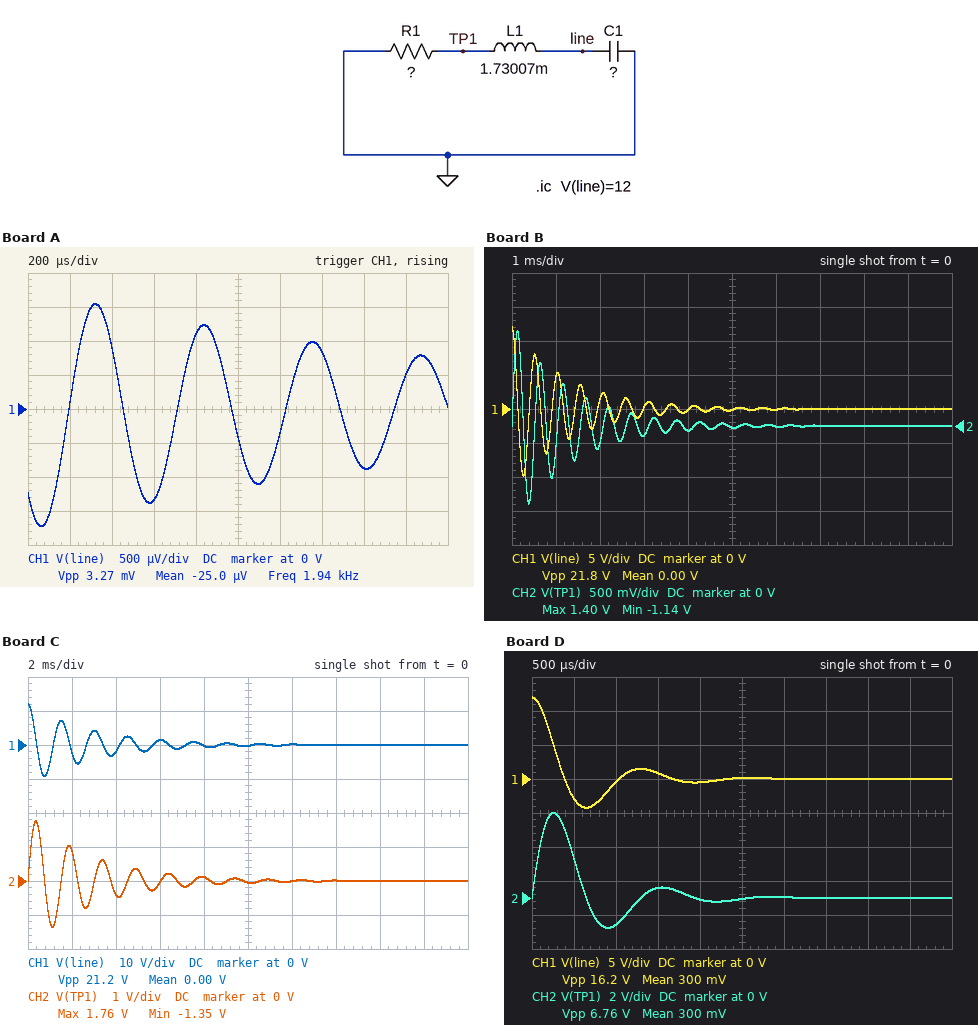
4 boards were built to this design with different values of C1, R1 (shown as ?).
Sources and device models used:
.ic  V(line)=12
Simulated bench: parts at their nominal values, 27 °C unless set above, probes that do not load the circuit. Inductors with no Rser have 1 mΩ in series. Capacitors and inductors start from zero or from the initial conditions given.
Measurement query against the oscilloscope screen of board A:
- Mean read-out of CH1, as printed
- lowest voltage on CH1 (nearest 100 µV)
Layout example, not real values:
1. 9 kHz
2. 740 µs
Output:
1. -25.0 µV
2. -1.7 mV
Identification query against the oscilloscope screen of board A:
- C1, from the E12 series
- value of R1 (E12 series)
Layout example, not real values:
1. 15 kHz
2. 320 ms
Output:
1. 3.9 µF
2. 1.5 Ω
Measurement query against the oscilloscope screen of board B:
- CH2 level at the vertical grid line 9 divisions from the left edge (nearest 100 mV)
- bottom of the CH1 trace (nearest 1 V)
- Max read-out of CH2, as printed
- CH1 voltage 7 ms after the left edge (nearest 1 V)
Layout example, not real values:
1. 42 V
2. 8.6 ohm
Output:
1. 0 V
2. -10 V
3. 1.40 V
4. 0 V
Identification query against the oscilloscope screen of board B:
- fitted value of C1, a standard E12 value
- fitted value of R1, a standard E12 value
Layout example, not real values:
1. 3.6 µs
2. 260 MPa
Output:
1. 3.9 µF
2. 2.7 Ω
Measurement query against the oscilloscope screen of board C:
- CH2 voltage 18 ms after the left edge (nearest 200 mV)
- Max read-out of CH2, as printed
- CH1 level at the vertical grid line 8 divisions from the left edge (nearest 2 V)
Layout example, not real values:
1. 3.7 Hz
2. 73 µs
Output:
1. 0 V
2. 1.76 V
3. 0 V
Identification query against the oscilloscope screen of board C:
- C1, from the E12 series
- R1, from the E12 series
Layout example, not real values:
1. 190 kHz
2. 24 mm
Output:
1. 33 µF
2. 1.2 Ω
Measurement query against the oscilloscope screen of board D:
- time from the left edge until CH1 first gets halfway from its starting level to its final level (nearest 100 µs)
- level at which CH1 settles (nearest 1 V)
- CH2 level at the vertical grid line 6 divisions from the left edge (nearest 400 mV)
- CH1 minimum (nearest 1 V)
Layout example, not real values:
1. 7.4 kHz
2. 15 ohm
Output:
1. 200 µs
2. 0 V
3. 0 V
4. -4 V
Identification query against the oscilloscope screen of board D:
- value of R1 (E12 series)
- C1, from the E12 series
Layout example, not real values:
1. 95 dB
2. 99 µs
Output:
1. 5.6 Ω
2. 22 µF
